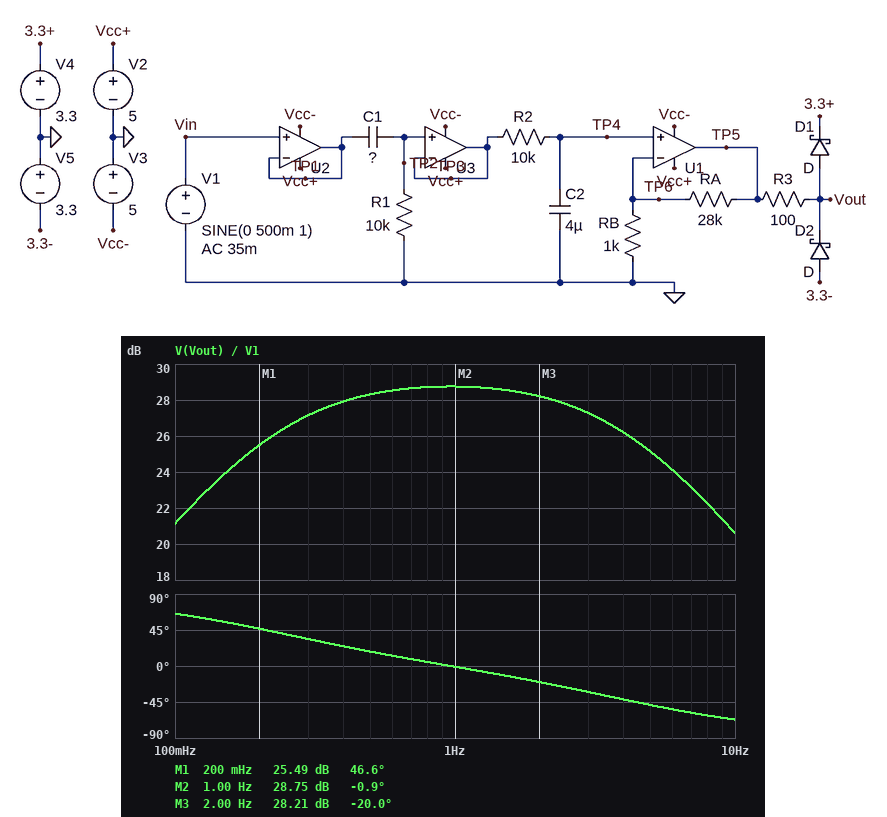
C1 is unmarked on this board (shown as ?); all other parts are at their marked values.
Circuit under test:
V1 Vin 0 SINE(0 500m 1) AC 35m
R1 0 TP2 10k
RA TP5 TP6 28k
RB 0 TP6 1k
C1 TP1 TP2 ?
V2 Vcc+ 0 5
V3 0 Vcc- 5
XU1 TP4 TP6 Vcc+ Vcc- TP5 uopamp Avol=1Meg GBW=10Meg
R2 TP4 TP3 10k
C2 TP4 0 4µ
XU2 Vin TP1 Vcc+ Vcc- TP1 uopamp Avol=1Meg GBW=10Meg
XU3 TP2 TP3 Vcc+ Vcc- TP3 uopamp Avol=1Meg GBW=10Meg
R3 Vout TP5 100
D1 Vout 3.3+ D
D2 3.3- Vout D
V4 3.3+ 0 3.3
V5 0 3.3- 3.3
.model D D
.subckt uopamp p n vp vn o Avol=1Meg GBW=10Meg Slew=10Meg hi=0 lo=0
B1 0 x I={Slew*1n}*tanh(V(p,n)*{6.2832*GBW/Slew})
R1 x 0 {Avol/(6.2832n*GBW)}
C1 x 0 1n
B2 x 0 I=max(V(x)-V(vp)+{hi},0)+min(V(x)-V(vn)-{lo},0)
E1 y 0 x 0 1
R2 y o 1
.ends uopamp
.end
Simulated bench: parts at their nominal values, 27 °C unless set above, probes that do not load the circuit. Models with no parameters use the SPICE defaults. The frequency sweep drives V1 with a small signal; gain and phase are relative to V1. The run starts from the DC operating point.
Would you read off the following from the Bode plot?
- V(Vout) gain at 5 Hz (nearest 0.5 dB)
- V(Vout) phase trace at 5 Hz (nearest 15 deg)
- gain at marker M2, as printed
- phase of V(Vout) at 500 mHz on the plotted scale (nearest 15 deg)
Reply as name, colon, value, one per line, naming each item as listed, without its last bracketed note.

V(Vout) gain at 5 Hz: 25.0 dB
V(Vout) phase trace at 5 Hz: -45 deg
gain at marker M2, as printed: 28.75 dB
phase of V(Vout) at 500 mHz on the plotted scale: 15 deg
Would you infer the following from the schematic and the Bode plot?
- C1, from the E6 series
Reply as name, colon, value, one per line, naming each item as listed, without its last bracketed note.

C1, from the E6 series: 68 µF
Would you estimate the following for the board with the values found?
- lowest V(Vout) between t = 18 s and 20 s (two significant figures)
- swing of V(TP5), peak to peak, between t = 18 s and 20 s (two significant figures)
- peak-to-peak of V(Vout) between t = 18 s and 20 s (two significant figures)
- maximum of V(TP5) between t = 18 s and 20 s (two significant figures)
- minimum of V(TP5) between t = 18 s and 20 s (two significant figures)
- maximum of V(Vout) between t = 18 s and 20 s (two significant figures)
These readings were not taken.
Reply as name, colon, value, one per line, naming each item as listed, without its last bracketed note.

lowest V(Vout) between t = 18 s and 20 s: -4.0 V
swing of V(TP5), peak to peak, between t = 18 s and 20 s: 10 V
peak-to-peak of V(Vout) between t = 18 s and 20 s: 8.0 V
maximum of V(TP5) between t = 18 s and 20 s: 5.0 V
minimum of V(TP5) between t = 18 s and 20 s: -5.0 V
maximum of V(Vout) between t = 18 s and 20 s: 4.0 V
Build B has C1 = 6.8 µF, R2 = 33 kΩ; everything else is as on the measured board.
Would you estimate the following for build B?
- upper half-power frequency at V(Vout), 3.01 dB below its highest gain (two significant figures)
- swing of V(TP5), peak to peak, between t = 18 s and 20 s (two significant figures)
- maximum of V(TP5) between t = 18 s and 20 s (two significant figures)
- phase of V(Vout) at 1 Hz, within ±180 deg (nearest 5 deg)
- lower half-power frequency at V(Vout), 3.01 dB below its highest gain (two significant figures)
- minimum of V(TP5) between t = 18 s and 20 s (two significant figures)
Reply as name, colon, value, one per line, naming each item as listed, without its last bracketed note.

upper half-power frequency at V(Vout), 3.01 dB below its highest gain: 4.2 Hz
swing of V(TP5), peak to peak, between t = 18 s and 20 s: 8.8 V
maximum of V(TP5) between t = 18 s and 20 s: 4.4 V
phase of V(Vout) at 1 Hz, within ±180 deg: 25 deg
lower half-power frequency at V(Vout), 3.01 dB below its highest gain: 670 mHz
minimum of V(TP5) between t = 18 s and 20 s: -4.4 V
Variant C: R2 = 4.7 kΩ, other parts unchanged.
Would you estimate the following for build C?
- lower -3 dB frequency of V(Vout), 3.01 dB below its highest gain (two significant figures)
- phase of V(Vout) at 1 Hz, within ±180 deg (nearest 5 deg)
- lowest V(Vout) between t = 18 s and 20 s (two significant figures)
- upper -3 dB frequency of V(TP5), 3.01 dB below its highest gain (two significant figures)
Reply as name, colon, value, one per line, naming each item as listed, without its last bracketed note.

lower -3 dB frequency of V(Vout), 3.01 dB below its highest gain: 220 mHz
phase of V(Vout) at 1 Hz, within ±180 deg: 5 deg
lowest V(Vout) between t = 18 s and 20 s: -4.0 V
upper -3 dB frequency of V(TP5), 3.01 dB below its highest gain: 8.9 Hz
